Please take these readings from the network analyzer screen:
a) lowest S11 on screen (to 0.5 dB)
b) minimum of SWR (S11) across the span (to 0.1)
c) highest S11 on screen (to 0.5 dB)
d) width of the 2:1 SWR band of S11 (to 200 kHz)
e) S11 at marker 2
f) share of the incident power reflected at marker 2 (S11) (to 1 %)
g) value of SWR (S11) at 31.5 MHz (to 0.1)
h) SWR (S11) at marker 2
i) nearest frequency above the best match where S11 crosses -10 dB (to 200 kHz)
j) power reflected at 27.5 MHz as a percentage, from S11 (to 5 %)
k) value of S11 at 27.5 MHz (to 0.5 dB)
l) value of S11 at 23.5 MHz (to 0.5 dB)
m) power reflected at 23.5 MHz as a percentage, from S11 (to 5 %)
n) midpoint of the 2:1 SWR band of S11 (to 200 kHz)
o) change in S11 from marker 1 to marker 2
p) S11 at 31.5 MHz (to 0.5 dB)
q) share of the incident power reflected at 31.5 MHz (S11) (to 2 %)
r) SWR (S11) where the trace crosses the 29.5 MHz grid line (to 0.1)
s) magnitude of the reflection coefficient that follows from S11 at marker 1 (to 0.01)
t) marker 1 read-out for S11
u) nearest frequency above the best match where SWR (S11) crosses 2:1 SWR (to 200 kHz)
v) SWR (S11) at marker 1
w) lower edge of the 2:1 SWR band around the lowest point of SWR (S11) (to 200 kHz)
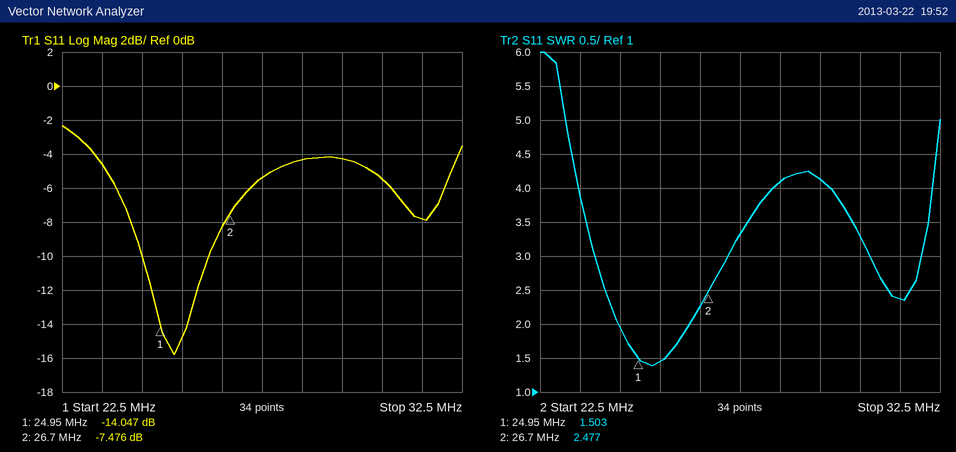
-16.0 dB
1.4
-2.5 dB
1.8 MHz
-7.476 dB
18 %
2.4
2.477
26.2 MHz
30 %
-5.5 dB
-4.5 dB
35 %
25.4 MHz
6.571 dB
-8.0 dB
16 %
4.1
0.20
-14.047 dB
26.2 MHz
1.503
24.4 MHz
